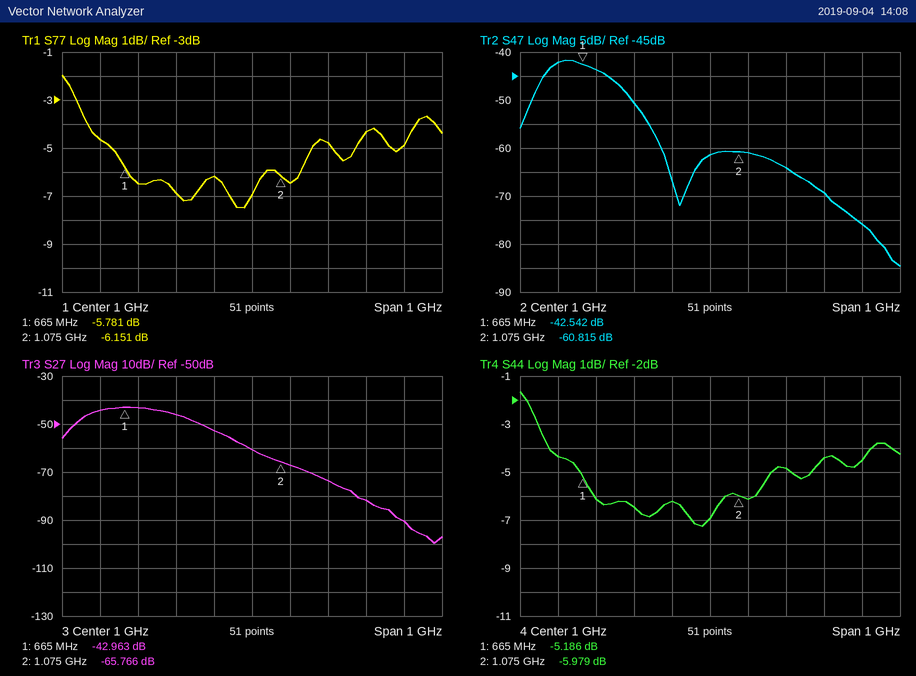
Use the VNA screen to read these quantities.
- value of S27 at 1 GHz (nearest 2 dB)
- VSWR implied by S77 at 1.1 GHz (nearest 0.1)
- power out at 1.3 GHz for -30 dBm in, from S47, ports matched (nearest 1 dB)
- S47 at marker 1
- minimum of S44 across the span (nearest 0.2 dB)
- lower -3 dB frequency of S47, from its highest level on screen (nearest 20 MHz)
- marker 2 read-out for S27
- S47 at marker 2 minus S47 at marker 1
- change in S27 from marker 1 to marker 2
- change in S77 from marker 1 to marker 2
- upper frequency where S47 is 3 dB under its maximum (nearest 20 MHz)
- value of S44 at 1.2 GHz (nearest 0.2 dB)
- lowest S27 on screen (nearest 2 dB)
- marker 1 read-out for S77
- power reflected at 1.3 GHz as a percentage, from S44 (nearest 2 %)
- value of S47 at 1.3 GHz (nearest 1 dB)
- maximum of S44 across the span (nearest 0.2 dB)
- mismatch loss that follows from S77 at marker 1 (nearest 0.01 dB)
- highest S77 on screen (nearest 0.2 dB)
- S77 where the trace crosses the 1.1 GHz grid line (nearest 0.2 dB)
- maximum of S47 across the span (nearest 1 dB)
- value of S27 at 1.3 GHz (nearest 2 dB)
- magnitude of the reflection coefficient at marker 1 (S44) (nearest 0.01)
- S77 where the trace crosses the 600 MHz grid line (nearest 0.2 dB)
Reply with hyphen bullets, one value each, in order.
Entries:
- -60 dB
- 2.8
- -99 dBm
- -42.542 dB
- -7.2 dB
- 560 MHz
- -65.766 dB
- -18.273 dB
- -22.803 dB
- -0.370 dB
- 720 MHz
- -4.8 dB
- -100 dB
- -5.781 dB
- 36 %
- -69 dB
- -1.6 dB
- 1.33 dB
- -2.0 dB
- -6.4 dB
- -42 dB
- -82 dB
- 0.55
- -4.6 dB
